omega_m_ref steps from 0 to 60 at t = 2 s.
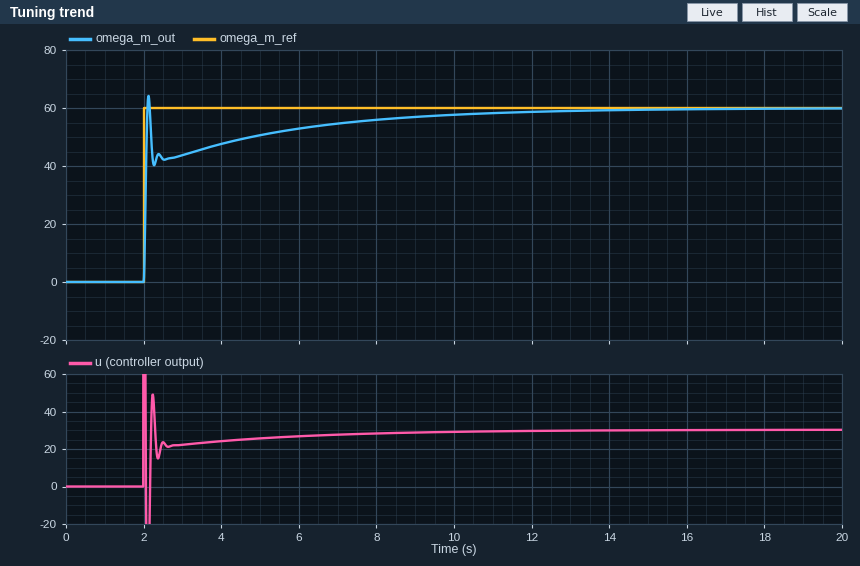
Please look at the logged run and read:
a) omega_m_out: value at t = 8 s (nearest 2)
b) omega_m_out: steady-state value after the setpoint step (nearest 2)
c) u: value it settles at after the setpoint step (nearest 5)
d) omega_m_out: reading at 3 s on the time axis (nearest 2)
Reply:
56
60
30
44
